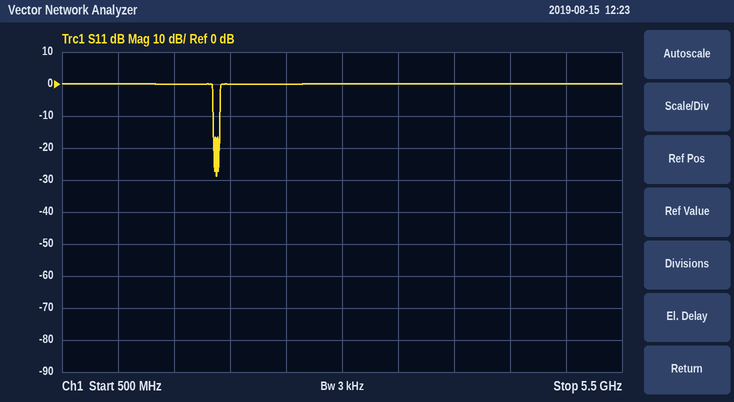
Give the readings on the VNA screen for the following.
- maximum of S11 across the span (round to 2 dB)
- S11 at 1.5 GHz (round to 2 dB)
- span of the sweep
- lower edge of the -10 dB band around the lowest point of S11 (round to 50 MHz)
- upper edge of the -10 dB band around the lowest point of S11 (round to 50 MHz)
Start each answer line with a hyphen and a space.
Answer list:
- 0 dB
- 0 dB
- 5 GHz
- 1.85 GHz
- 1.90 GHz
